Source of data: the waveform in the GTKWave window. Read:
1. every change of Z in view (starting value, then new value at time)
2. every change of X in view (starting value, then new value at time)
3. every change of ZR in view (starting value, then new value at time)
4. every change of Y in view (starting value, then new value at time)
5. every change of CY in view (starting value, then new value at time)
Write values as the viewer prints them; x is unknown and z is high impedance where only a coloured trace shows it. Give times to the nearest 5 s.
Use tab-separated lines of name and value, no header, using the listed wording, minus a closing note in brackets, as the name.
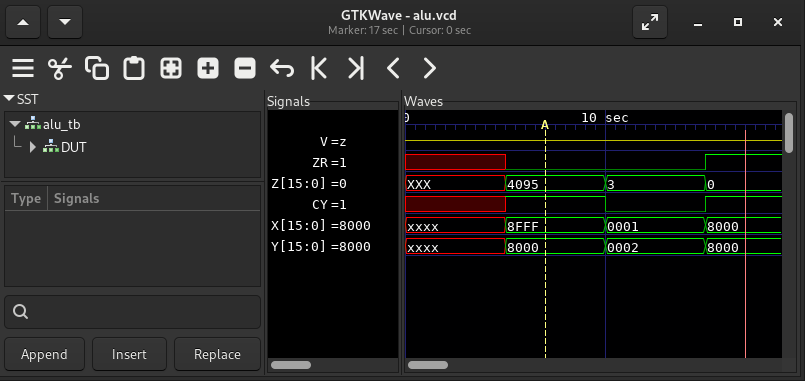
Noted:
every change of Z in view	XXX, 4095 at 5 s, 3 at 10 s, 0 at 15 s
every change of X in view	xxxx, 8FFF at 5 s, 0001 at 10 s, 8000 at 15 s
every change of ZR in view	x, 0 at 5 s, 1 at 15 s
every change of Y in view	xxxx, 8000 at 5 s, 0002 at 10 s, 8000 at 15 s
every change of CY in view	x, 1 at 5 s, 0 at 10 s, 1 at 15 s
